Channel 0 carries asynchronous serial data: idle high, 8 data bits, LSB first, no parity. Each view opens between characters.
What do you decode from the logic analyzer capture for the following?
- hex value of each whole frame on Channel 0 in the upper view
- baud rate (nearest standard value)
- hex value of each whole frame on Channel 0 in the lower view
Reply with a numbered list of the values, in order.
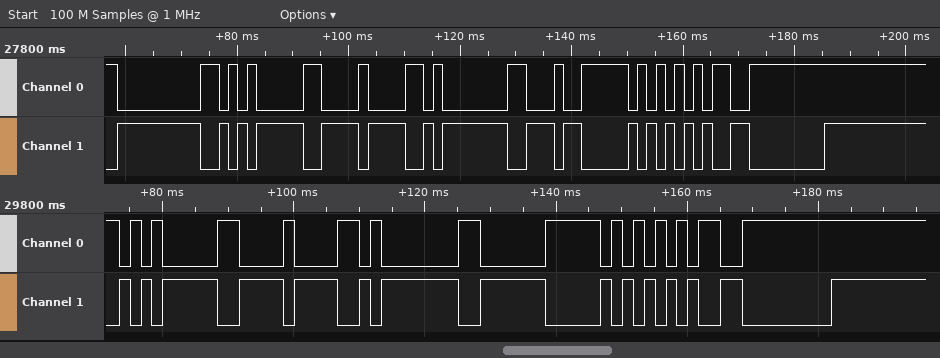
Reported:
1. 00, 05, 08, 01, E4, 55, FE
2. 600 baud
3. 05, 08, 01, E0, 55, FE
